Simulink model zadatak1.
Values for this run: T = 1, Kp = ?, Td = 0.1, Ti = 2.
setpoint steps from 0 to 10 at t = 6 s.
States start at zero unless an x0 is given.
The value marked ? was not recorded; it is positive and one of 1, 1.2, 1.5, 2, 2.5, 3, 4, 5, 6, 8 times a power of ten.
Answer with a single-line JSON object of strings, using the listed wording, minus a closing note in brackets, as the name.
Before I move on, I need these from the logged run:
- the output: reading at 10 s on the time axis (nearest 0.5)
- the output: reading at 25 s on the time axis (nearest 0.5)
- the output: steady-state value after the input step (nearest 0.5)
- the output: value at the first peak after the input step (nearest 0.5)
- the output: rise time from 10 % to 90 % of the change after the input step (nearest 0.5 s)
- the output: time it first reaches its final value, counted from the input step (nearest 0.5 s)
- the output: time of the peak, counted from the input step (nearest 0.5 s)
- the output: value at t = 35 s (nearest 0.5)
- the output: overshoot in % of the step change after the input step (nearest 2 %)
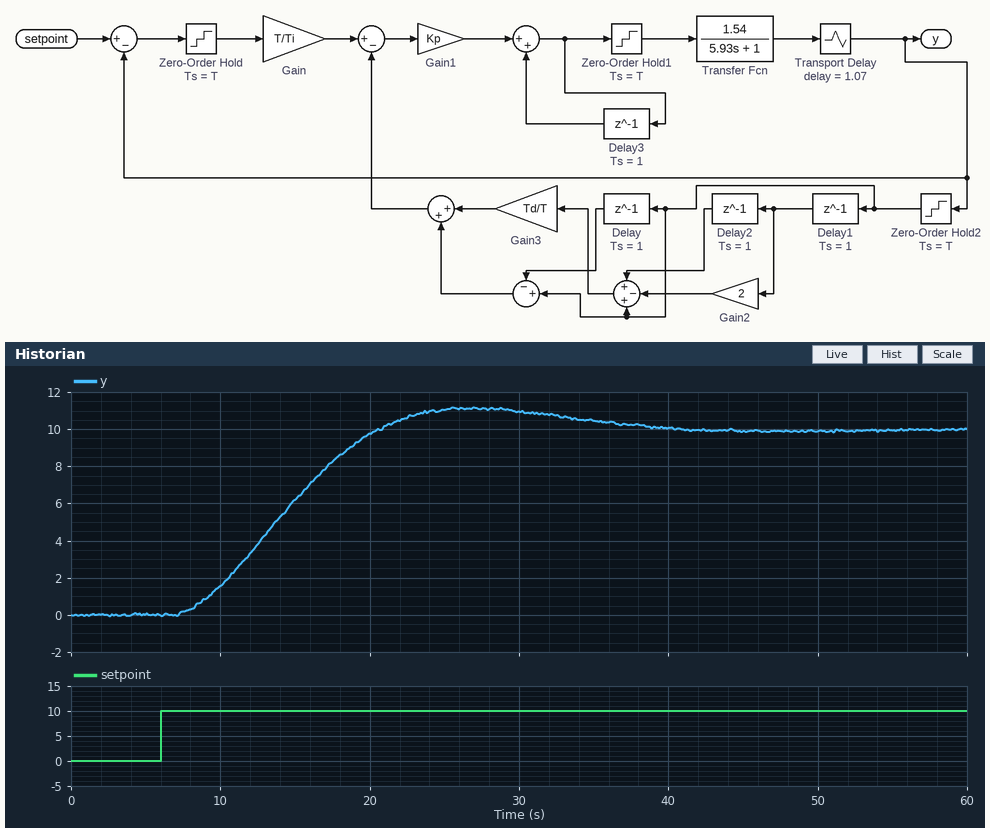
{"the output: reading at 10 s on the time axis": "1.5", "the output: reading at 25 s on the time axis": "11.0", "the output: steady-state value after the input step": "10.0", "the output: value at the first peak after the input step": "11.0", "the output: rise time from 10 % to 90 % of the change after the input step": "9.5 s", "the output: time it first reaches its final value, counted from the input step": "14.5 s", "the output: time of the peak, counted from the input step": "21.0 s", "the output: value at t = 35 s": "10.5", "the output: overshoot in % of the step change after the input step": "12 %"}
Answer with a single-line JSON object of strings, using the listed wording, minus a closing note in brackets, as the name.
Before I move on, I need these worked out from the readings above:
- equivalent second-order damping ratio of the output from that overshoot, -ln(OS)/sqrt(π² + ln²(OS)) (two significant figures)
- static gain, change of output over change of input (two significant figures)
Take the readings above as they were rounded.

{"equivalent second-order damping ratio of the output from that overshoot, -ln(OS)/sqrt(π² + ln²(OS))": "0.56", "static gain, change of output over change of input": "1.0"}
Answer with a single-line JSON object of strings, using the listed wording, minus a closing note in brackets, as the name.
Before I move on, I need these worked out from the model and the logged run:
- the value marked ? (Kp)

{"the value marked ?": "0.25"}
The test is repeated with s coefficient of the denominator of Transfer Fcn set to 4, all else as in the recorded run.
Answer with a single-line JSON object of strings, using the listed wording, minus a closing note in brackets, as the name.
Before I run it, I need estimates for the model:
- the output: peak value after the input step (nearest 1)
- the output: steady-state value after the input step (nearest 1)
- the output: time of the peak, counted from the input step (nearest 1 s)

{"the output: peak value after the input step": "10", "the output: steady-state value after the input step": "10", "the output: time of the peak, counted from the input step": "19 s"}
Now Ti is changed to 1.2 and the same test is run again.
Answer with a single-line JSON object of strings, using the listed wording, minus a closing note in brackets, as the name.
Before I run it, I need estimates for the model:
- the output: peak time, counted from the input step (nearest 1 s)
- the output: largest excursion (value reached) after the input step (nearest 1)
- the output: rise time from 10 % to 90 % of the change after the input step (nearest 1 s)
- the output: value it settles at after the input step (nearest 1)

{"the output: peak time, counted from the input step": "15 s", "the output: largest excursion (value reached) after the input step": "13", "the output: rise time from 10 % to 90 % of the change after the input step": "6 s", "the output: value it settles at after the input step": "10"}
